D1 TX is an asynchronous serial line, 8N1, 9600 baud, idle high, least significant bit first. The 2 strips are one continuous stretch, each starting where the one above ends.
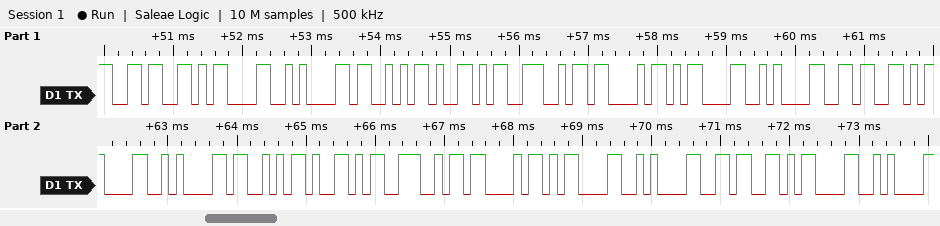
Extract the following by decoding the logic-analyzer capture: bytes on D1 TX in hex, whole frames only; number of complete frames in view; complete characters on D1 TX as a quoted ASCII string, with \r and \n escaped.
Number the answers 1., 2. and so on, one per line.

1. 36 0D 0A 53 59 4E 43 0D 0A 36 0D 0A 53 59 4E 43 0D 0A 36 0D 0A
2. 21
3. "6\r\nSYNC\r\n6\r\nSYNC\r\n6\r\n"
